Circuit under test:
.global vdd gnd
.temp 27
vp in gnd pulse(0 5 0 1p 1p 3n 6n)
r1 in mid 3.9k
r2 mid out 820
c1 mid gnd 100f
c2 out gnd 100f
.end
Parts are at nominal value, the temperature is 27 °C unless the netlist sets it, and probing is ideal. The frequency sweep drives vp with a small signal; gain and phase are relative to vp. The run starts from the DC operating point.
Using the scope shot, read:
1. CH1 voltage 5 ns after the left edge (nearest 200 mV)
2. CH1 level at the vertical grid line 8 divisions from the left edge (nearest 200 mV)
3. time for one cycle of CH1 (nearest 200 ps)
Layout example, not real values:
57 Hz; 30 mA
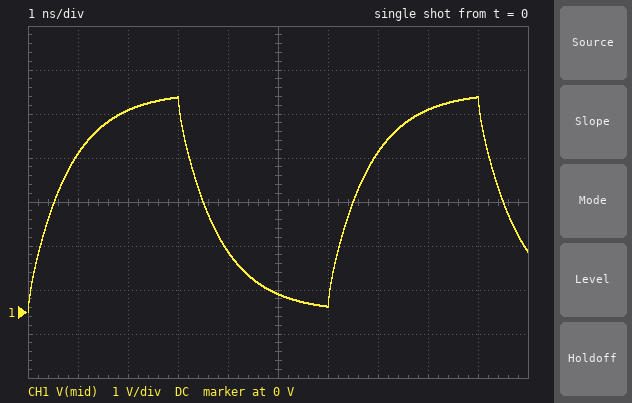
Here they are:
400 mV; 4.6 V; 6.0 ns
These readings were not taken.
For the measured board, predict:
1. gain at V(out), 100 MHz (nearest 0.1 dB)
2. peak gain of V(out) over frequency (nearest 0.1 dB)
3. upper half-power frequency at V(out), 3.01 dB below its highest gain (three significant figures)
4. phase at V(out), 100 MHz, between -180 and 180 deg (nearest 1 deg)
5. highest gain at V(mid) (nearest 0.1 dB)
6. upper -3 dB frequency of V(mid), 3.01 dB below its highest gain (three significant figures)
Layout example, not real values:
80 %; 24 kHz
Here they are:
-1.0 dB; 0 dB; 193 MHz; -29 deg; 0 dB; 195 MHz
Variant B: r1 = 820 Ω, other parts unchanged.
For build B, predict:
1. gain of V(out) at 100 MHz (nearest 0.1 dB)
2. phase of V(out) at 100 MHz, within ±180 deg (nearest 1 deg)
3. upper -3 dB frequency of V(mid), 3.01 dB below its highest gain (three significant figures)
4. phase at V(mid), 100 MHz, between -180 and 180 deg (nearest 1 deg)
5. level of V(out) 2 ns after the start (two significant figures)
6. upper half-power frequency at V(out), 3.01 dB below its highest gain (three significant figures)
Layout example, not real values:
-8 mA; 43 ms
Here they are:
-0.1 dB; -9 deg; 852 MHz; -6 deg; 5.0 V; 726 MHz
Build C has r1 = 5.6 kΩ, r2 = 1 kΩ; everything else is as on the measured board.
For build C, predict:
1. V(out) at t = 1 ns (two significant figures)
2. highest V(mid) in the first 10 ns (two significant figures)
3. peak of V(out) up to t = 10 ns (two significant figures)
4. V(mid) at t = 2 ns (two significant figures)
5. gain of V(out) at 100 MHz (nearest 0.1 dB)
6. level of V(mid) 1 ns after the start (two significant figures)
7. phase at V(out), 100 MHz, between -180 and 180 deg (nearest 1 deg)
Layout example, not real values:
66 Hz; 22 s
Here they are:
2.8 V; 4.7 V; 4.6 V; 4.1 V; -1.9 dB; 3.0 V; -38 deg
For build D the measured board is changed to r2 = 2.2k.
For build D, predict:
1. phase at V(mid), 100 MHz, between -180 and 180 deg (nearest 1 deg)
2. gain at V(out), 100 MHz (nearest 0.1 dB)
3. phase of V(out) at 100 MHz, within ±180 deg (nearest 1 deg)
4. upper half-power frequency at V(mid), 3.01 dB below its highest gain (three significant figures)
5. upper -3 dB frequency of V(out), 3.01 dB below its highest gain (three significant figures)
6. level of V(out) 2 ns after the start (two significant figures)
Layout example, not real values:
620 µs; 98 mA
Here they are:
-25 deg; -1.2 dB; -33 deg; 185 MHz; 174 MHz; 4.4 V
